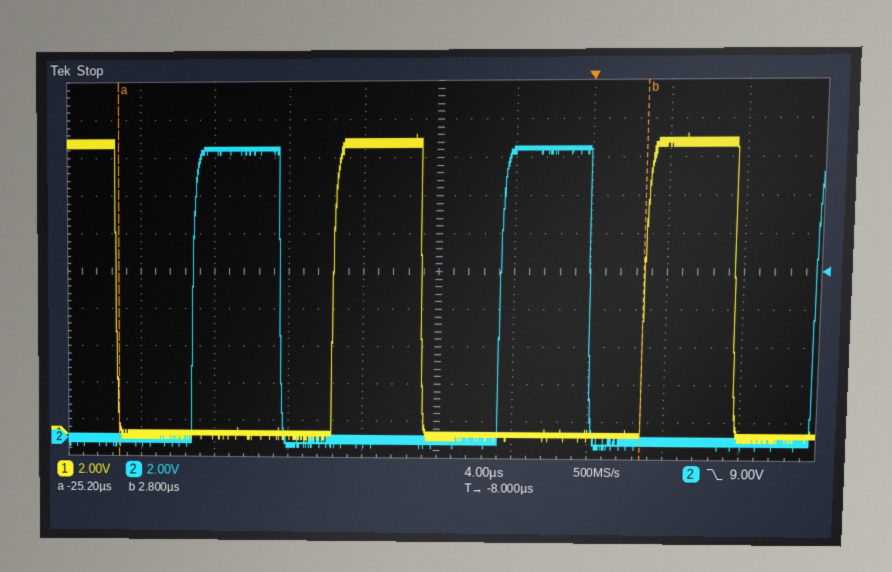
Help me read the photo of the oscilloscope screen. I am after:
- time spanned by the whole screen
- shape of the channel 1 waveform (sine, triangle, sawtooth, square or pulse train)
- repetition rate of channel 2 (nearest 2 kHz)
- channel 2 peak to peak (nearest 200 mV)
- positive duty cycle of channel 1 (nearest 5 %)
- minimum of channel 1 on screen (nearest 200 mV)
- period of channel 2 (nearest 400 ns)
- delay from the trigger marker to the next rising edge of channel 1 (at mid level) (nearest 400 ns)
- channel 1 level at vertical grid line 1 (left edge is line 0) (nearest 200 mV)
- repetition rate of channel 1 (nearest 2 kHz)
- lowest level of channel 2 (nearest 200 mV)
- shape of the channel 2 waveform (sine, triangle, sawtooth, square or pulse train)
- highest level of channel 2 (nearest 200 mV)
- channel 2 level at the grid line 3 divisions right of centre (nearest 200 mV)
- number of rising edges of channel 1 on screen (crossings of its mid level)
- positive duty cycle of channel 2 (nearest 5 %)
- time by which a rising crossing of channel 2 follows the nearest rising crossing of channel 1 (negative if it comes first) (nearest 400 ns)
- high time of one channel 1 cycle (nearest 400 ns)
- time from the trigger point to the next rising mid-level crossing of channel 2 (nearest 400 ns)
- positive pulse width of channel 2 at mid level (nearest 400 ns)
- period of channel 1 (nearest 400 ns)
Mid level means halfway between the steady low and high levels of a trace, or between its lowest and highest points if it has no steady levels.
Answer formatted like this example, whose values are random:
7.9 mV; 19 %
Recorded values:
40 µs; pulse train; 60 kHz; 16.0 V; 30 %; -200 mV; 16.4 µs; 2.8 µs; 0.0 V; 60 kHz; -400 mV; pulse train; 15.6 V; 0.0 V; 2; 30 %; -7.6 µs; 4.8 µs; 11.6 µs; 4.8 µs; 16.4 µs
